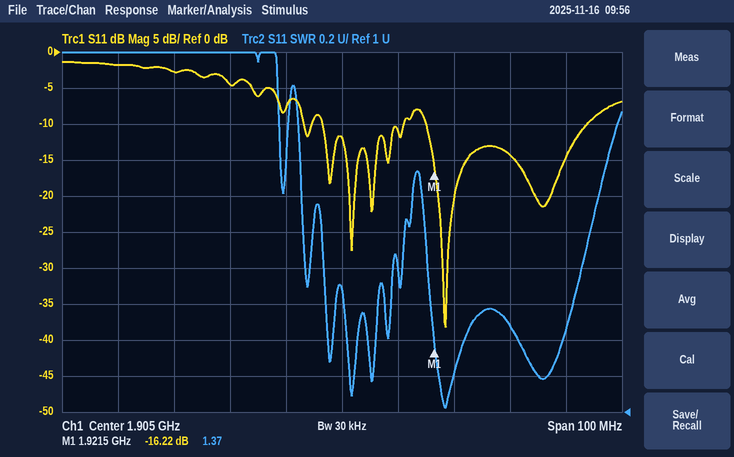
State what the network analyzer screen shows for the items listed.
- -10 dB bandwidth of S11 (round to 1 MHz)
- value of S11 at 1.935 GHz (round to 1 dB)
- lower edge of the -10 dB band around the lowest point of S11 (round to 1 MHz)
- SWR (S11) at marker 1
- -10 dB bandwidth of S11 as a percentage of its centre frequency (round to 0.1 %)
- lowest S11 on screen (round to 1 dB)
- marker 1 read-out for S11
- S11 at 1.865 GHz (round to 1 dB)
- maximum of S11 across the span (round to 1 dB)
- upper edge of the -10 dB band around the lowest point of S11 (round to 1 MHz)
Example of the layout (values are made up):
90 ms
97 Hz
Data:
29 MHz
-14 dB
1.920 GHz
1.37
1.5 %
-38 dB
-16.22 dB
-2 dB
-1 dB
1.949 GHz
